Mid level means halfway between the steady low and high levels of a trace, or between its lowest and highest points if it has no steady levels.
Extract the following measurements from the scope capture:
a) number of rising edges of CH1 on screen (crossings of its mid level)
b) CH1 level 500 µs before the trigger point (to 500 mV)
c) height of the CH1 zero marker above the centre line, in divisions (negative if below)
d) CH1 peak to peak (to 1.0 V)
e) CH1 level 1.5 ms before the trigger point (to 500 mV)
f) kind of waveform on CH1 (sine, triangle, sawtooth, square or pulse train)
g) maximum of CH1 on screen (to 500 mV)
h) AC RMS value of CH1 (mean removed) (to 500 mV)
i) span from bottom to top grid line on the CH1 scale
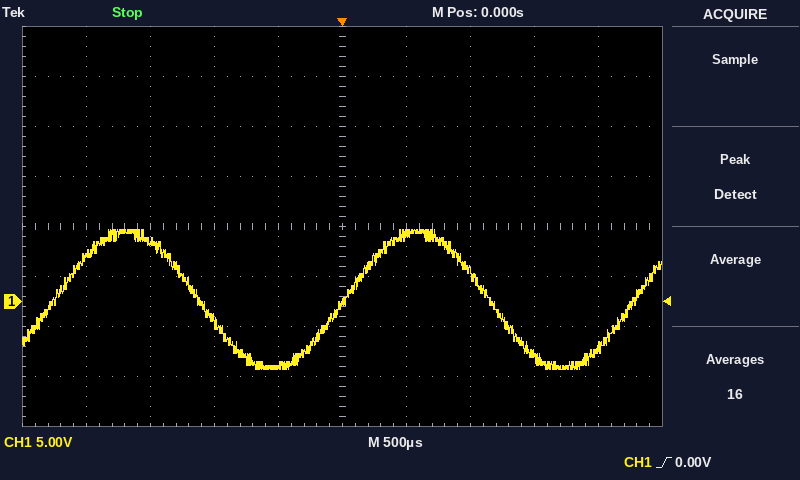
3
-6.5 V
-1.5 div
14.0 V
6.0 V
sine
7.0 V
5.0 V
40 V
